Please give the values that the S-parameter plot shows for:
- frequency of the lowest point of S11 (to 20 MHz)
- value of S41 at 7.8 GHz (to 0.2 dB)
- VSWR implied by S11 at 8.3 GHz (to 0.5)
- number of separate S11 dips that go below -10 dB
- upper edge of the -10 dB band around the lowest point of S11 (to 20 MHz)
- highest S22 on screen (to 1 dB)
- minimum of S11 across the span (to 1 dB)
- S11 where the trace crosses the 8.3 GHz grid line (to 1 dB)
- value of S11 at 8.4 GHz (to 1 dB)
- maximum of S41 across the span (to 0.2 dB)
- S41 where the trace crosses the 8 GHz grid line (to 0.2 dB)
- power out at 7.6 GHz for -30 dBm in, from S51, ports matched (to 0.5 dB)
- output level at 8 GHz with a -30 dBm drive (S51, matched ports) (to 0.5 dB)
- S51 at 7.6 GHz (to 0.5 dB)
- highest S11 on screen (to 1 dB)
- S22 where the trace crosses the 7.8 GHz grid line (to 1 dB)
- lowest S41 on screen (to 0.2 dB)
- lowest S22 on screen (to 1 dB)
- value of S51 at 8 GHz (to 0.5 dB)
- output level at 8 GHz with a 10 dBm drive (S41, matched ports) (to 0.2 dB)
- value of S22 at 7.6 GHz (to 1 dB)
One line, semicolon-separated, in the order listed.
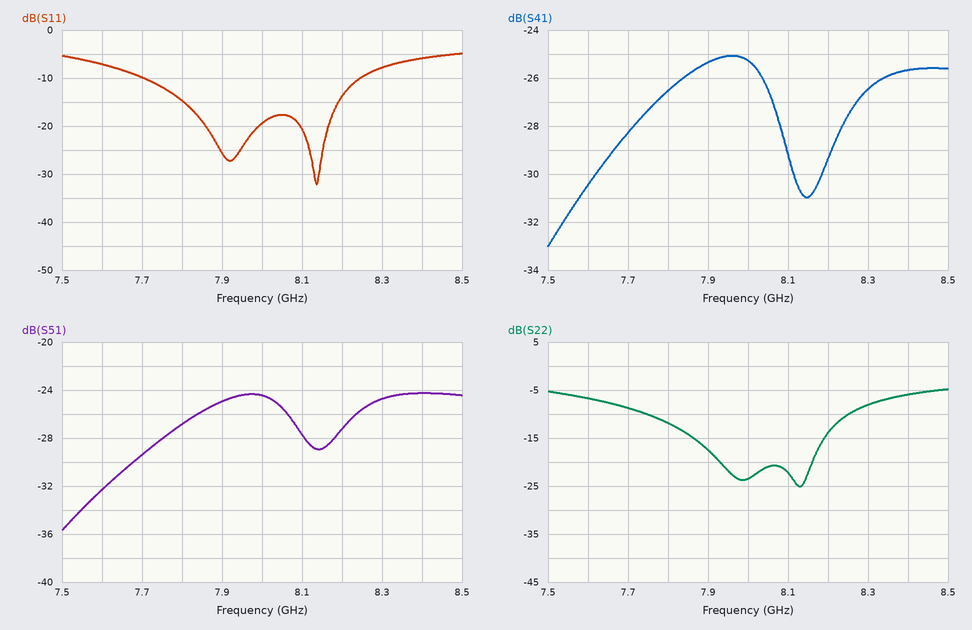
8.14 GHz; -26.6 dB; 2.5; 2; 8.24 GHz; -5 dB; -32 dB; -8 dB; -6 dB; -25.0 dB; -25.2 dB; -62.5 dBm; -54.5 dBm; -32.5 dB; -5 dB; -12 dB; -33.0 dB; -25 dB; -24.5 dB; -15.2 dBm; -7 dB
